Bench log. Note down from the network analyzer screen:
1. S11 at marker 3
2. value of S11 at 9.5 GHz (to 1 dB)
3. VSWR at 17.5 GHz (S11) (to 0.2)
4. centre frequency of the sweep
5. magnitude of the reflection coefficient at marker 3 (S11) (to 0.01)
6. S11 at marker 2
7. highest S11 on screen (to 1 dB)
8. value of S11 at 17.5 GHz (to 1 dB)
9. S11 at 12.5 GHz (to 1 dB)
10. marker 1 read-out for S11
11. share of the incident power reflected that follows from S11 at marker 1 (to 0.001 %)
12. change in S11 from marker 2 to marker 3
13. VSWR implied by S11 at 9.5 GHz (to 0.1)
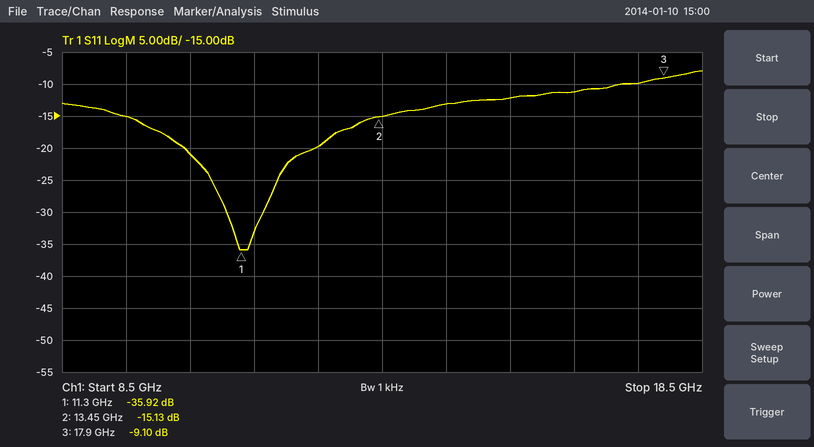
-9.10 dB
-15 dB
2.0
13.5 GHz
0.35
-15.13 dB
-8 dB
-10 dB
-20 dB
-35.92 dB
0.026 %
6.03 dB
1.4
